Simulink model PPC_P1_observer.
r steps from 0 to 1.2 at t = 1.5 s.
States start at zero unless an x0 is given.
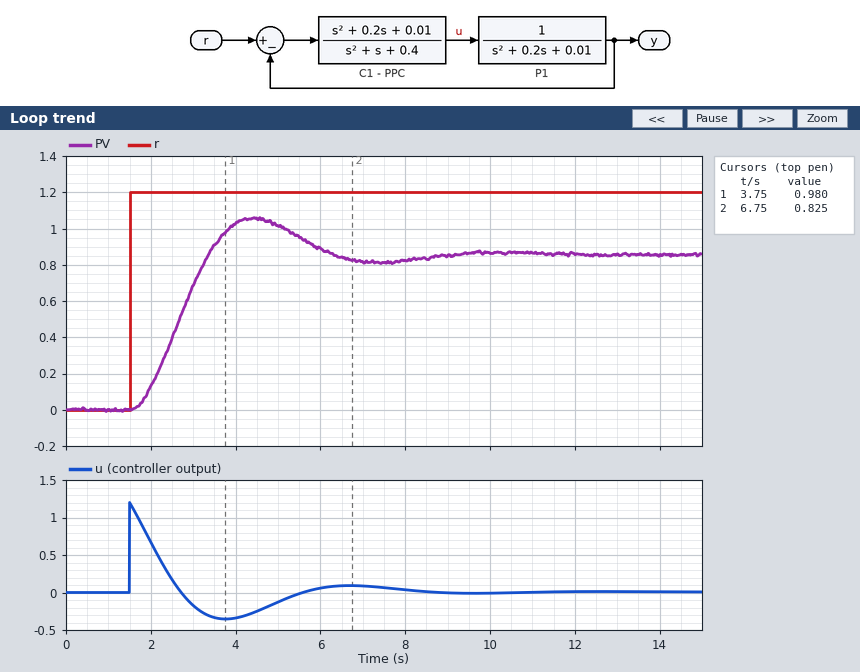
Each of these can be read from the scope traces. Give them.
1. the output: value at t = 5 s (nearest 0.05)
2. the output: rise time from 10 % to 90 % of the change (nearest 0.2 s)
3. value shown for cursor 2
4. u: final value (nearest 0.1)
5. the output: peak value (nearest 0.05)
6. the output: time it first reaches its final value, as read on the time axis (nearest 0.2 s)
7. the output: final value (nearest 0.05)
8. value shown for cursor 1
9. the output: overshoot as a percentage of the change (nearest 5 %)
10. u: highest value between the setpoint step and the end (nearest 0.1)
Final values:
1.00
1.2 s
0.825
0.0
1.05
3.4 s
0.85
0.980
25 %
1.2
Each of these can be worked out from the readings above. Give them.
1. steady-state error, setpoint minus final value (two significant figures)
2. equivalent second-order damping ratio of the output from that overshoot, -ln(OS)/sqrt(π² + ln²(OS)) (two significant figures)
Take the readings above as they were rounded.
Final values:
0.35
0.40
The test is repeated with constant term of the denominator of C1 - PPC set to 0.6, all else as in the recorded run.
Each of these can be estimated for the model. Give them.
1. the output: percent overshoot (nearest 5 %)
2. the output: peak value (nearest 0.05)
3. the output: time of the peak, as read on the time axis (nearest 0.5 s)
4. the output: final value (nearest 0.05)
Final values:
25 %
0.95
4.0 s
0.75
